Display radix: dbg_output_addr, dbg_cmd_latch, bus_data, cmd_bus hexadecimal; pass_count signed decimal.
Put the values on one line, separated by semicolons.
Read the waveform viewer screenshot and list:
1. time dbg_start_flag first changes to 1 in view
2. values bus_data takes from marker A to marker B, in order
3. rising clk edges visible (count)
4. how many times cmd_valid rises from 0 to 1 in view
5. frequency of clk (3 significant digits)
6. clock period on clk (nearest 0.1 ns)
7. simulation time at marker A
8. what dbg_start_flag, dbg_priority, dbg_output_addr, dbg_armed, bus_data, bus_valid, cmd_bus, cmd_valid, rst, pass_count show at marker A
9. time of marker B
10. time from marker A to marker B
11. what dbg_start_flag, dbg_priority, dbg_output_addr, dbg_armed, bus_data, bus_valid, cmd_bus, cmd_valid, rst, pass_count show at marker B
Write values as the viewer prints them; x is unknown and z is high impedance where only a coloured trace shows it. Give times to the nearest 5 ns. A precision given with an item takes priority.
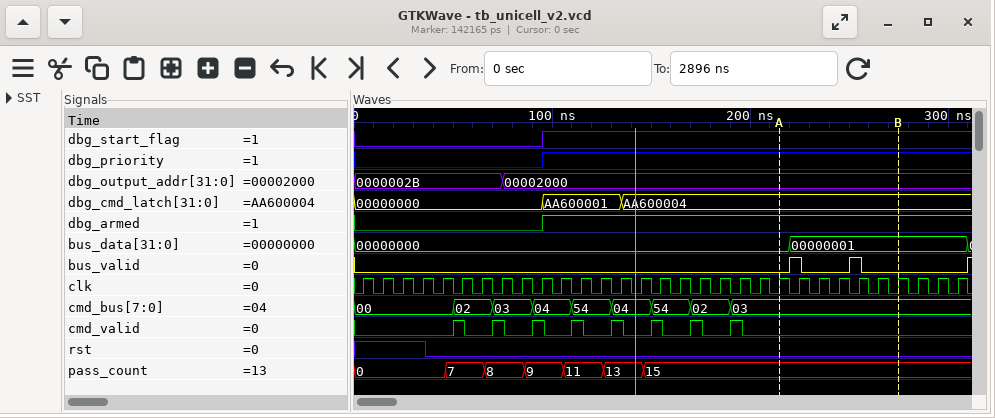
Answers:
95 ns; 00000000, 00000001; 31; 8; 100 MHz; 10 ns; 215 ns; dbg_start_flag=1, dbg_priority=1, dbg_output_addr=00002000, dbg_armed=1, bus_data=00000000, bus_valid=0, cmd_bus=03, cmd_valid=0, rst=0, pass_count=15; 275 ns; 60 ns; dbg_start_flag=1, dbg_priority=1, dbg_output_addr=00002000, dbg_armed=1, bus_data=00000001, bus_valid=0, cmd_bus=03, cmd_valid=0, rst=0, pass_count=15
